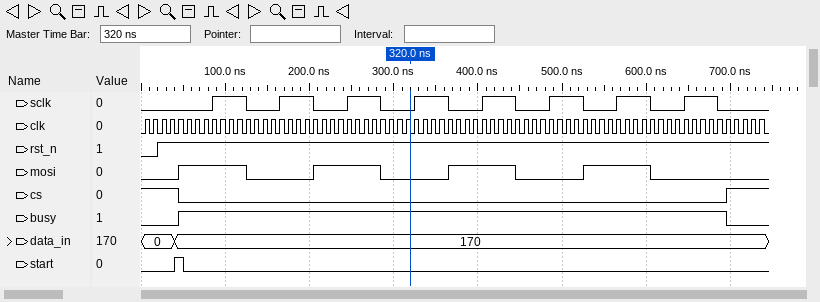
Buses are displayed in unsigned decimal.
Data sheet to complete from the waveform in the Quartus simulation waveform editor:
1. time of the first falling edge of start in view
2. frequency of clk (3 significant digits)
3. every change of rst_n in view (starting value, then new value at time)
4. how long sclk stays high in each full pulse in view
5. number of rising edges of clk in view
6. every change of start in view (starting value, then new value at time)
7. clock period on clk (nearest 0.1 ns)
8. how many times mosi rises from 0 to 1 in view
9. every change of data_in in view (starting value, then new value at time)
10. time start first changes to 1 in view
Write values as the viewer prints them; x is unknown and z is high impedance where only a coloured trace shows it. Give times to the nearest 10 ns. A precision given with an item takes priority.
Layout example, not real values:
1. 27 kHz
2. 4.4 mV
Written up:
1. 50 ns
2. 100 MHz
3. 0, 1 at 20 ns
4. 40 ns, 40 ns, 40 ns, 40 ns, 40 ns, 40 ns, 40 ns, 40 ns
5. 74
6. 0, 1 at 40 ns, 0 at 50 ns
7. 10 ns
8. 4
9. 0, 170 at 40 ns
10. 40 ns
